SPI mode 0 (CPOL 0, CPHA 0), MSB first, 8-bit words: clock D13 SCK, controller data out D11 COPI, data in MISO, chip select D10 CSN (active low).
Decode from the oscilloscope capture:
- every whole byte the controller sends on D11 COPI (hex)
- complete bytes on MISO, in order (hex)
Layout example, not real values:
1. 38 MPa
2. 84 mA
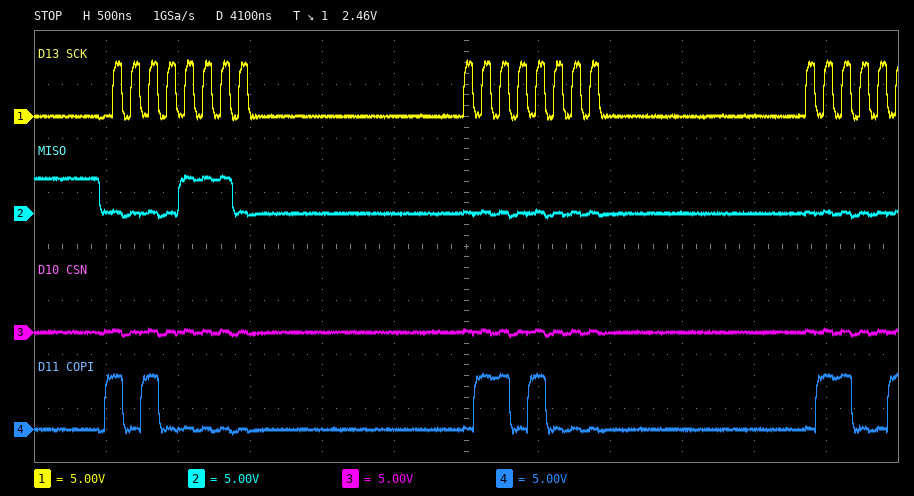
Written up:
1. 0xA0 0x68
2. 0x0E 0x00
